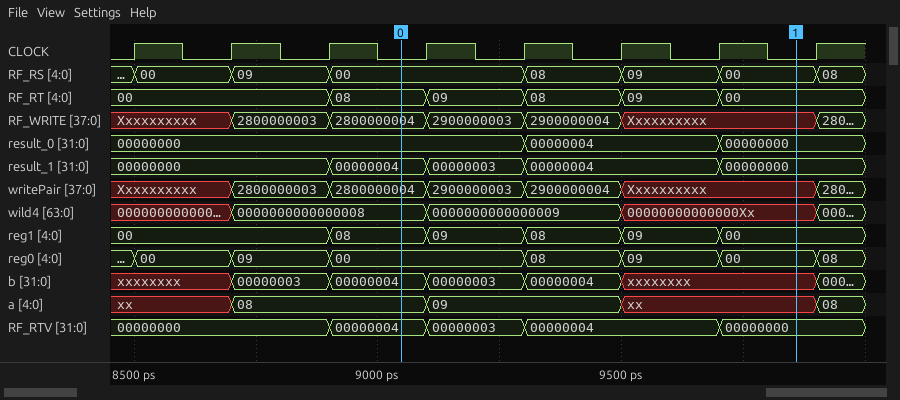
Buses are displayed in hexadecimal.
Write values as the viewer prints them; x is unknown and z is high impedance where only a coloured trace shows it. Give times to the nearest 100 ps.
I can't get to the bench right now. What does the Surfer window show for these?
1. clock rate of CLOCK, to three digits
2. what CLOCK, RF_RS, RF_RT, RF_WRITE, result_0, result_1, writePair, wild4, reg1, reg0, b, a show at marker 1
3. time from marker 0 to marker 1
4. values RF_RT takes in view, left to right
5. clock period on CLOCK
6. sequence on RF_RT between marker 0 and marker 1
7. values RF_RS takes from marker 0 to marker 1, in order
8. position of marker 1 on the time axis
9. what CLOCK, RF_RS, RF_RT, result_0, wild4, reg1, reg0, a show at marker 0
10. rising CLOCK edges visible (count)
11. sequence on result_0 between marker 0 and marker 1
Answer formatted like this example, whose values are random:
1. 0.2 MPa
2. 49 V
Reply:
1. 5.00 GHz
2. CLOCK=0, RF_RS=00, RF_RT=00, RF_WRITE=Xxxxxxxxxx, result_0=00000000, result_1=00000000, writePair=Xxxxxxxxxx, wild4=00000000000000Xx, reg1=00, reg0=00, b=xxxxxxxx, a=xx
3. 800 ps
4. 00, 08, 09, 08, 09, 00
5. 200 ps
6. 08, 09, 08, 09, 00
7. 00, 08, 09, 00
8. 9900 ps
9. CLOCK=0, RF_RS=00, RF_RT=08, result_0=00000000, wild4=0000000000000008, reg1=08, reg0=00, a=08
10. 8
11. 00000000, 00000004, 00000000
